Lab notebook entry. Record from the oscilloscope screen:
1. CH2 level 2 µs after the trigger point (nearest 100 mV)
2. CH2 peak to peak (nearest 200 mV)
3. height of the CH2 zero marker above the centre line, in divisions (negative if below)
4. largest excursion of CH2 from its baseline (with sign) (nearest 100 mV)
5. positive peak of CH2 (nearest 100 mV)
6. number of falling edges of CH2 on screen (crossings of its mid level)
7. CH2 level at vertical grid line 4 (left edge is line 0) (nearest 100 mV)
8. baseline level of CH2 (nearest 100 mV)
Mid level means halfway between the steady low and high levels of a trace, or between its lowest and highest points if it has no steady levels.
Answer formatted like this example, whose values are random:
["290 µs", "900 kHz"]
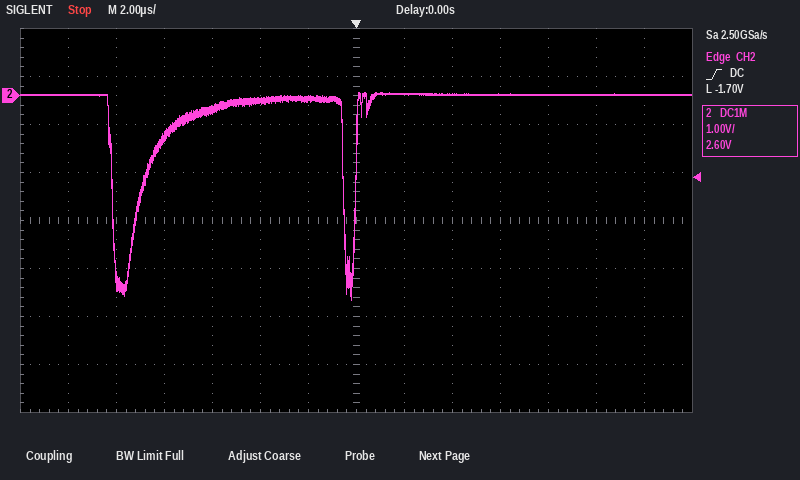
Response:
["0.0 V", "4.4 V", "+2.6 div", "-4.3 V", "100 mV", "2", "-300 mV", "0.0 V"]
